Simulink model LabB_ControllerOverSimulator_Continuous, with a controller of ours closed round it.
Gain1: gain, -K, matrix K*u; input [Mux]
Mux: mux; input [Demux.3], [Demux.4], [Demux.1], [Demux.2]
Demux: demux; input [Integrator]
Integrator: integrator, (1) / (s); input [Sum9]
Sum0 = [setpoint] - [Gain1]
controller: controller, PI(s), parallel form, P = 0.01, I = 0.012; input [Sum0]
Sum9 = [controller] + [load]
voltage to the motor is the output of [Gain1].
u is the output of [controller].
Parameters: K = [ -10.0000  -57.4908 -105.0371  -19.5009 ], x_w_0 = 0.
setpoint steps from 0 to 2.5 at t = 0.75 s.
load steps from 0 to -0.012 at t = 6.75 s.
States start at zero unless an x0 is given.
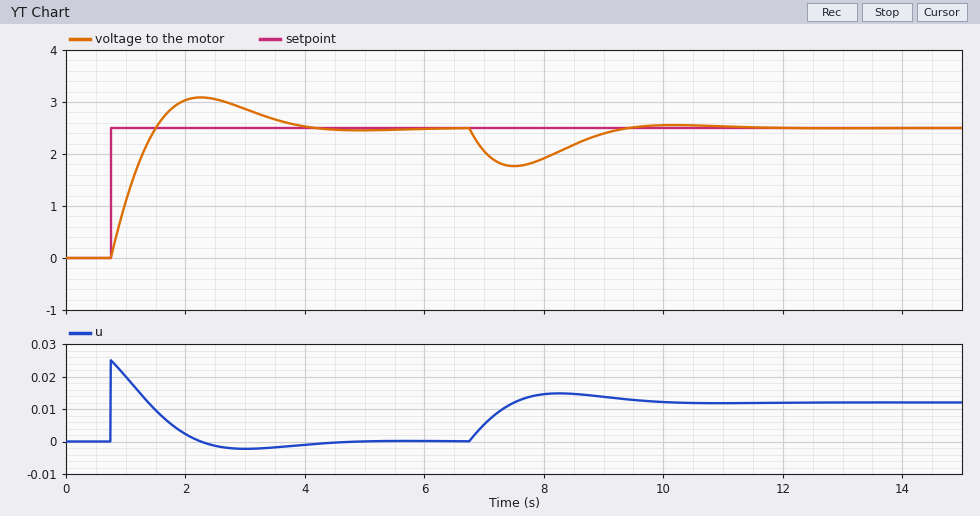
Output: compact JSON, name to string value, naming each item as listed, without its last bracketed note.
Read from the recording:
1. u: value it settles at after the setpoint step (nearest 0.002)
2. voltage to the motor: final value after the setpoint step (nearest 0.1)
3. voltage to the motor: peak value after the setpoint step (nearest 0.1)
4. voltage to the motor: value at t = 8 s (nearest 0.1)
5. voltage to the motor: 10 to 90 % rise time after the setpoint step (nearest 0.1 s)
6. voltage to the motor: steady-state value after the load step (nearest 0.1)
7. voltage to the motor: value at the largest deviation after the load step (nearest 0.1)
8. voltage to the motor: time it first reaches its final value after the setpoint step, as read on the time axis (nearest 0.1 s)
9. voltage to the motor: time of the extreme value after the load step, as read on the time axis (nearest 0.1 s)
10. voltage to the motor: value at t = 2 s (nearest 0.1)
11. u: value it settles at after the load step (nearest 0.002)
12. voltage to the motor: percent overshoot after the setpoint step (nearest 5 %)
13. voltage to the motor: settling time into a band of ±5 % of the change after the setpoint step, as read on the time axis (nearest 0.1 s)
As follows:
{"u: value it settles at after the setpoint step": "0.000", "voltage to the motor: final value after the setpoint step": "2.5", "voltage to the motor: peak value after the setpoint step": "3.1", "voltage to the motor: value at t = 8 s": "1.9", "voltage to the motor: 10 to 90 % rise time after the setpoint step": "0.6 s", "voltage to the motor: steady-state value after the load step": "2.5", "voltage to the motor: value at the largest deviation after the load step": "1.8", "voltage to the motor: time it first reaches its final value after the setpoint step, as read on the time axis": "1.5 s", "voltage to the motor: time of the extreme value after the load step, as read on the time axis": "7.5 s", "voltage to the motor: value at t = 2 s": "3.0", "u: value it settles at after the load step": "0.012", "voltage to the motor: percent overshoot after the setpoint step": "25 %", "voltage to the motor: settling time into a band of ±5 % of the change after the setpoint step, as read on the time axis": "3.6 s"}
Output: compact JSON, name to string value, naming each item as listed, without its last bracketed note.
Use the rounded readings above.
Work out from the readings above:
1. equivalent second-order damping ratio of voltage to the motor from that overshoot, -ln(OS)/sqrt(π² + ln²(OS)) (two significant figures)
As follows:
{"equivalent second-order damping ratio of voltage to the motor from that overshoot, -ln(OS)/sqrt(π² + ln²(OS))": "0.40"}
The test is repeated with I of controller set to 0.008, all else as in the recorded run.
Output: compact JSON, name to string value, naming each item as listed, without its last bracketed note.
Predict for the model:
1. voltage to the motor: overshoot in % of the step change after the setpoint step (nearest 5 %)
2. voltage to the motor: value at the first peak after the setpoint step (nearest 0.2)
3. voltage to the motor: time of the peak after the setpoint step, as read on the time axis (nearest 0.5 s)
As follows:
{"voltage to the motor: overshoot in % of the step change after the setpoint step": "20 %", "voltage to the motor: value at the first peak after the setpoint step": "3.0", "voltage to the motor: time of the peak after the setpoint step, as read on the time axis": "2.5 s"}
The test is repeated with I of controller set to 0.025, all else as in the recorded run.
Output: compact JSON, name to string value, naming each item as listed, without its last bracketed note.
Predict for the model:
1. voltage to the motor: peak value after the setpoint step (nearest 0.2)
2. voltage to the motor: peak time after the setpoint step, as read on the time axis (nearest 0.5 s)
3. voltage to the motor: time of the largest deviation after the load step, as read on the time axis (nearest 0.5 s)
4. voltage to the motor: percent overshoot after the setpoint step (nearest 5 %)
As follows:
{"voltage to the motor: peak value after the setpoint step": "3.4", "voltage to the motor: peak time after the setpoint step, as read on the time axis": "2.0 s", "voltage to the motor: time of the largest deviation after the load step, as read on the time axis": "7.5 s", "voltage to the motor: percent overshoot after the setpoint step": "35 %"}
